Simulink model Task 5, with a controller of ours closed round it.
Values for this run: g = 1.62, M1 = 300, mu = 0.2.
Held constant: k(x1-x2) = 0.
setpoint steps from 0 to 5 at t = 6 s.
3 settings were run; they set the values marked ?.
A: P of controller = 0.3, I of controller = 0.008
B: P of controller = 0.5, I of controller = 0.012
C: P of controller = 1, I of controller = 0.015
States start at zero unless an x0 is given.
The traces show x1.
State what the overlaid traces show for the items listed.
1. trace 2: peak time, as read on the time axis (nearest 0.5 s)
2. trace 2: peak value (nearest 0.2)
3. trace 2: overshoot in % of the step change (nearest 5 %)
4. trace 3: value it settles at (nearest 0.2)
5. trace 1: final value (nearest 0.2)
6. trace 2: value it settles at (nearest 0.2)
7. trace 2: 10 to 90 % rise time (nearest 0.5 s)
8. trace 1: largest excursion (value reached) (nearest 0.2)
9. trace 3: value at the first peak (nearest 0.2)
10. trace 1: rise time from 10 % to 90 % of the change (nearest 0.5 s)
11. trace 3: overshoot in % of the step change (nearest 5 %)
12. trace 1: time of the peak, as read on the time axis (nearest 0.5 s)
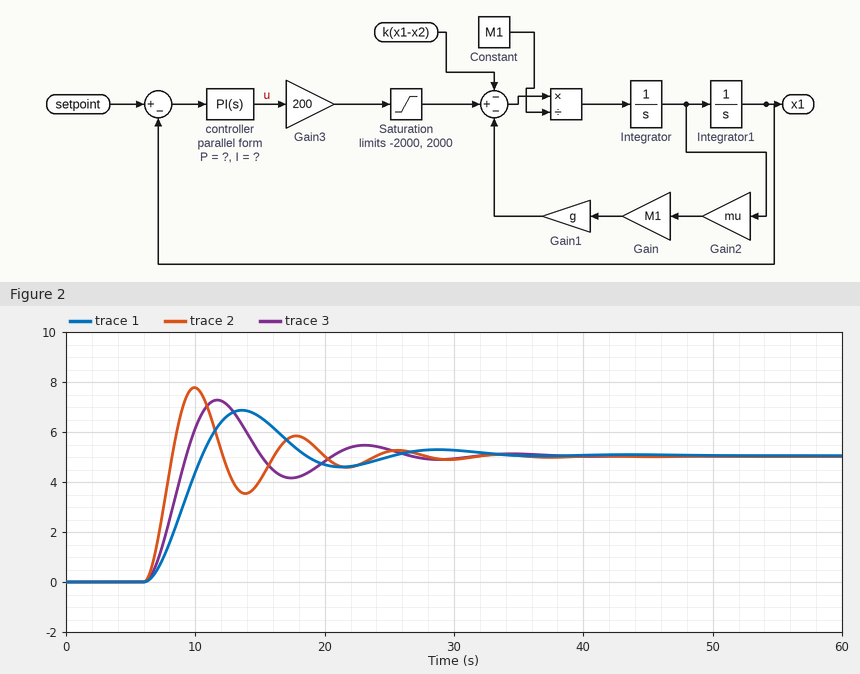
10.0 s
7.8
55 %
5.0
5.0
5.0
1.5 s
6.8
7.2
3.0 s
45 %
13.5 s
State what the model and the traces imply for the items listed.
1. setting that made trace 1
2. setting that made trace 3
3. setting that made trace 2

A
B
C
